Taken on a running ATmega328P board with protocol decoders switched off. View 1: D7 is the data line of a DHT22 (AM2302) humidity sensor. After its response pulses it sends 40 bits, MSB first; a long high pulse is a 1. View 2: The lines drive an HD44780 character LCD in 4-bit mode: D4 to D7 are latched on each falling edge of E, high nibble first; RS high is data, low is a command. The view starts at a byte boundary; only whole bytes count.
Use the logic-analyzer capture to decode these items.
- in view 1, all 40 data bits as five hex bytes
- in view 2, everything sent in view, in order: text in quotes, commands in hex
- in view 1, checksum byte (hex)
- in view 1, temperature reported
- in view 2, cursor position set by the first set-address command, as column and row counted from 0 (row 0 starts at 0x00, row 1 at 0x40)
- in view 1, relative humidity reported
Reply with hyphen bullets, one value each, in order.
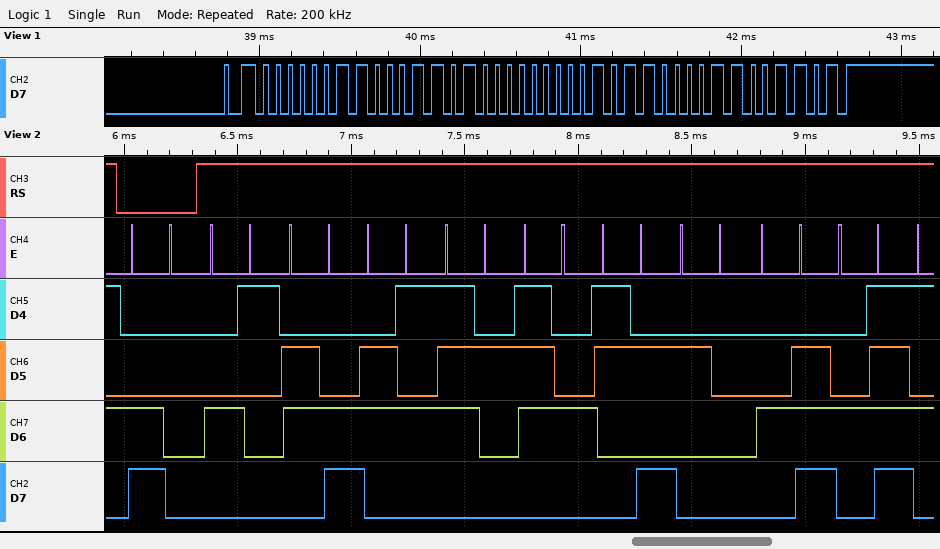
- 03 1A 00 B0 CD
- 0xC0 "Alert: NO"
- 0xCD
- 17.6 °C
- column 0, row 1
- 79.4 %
